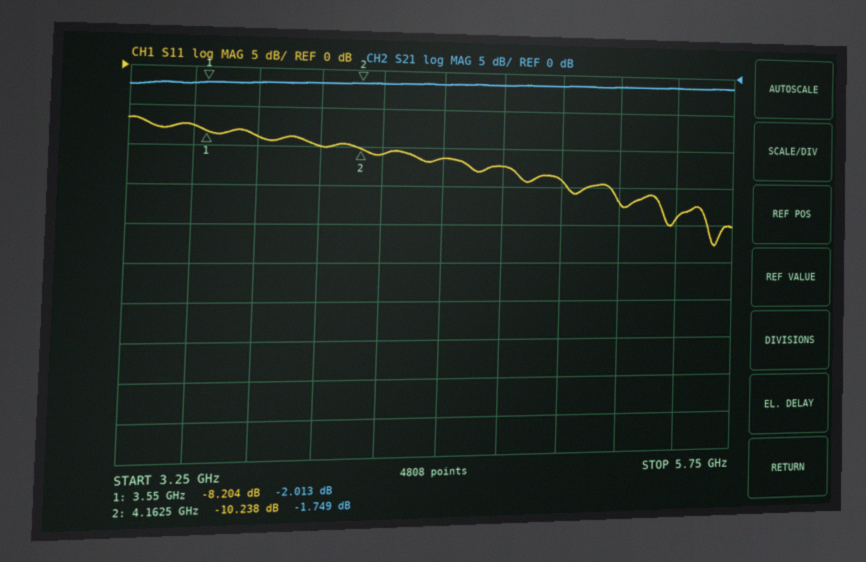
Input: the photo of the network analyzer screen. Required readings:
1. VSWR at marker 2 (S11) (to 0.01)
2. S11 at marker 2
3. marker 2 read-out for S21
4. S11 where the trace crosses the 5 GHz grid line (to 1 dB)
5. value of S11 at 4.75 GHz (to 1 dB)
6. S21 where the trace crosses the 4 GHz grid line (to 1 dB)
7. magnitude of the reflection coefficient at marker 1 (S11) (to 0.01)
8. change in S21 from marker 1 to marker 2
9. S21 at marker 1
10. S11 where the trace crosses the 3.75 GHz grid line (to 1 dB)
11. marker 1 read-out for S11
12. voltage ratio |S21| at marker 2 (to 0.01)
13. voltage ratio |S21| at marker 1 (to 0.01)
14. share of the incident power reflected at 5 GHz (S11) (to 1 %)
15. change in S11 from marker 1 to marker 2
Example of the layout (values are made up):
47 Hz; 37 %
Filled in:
1.89; -10.238 dB; -1.749 dB; -14 dB; -12 dB; -2 dB; 0.39; 0.264 dB; -2.013 dB; -9 dB; -8.204 dB; 0.82; 0.79; 4 %; -2.034 dB
